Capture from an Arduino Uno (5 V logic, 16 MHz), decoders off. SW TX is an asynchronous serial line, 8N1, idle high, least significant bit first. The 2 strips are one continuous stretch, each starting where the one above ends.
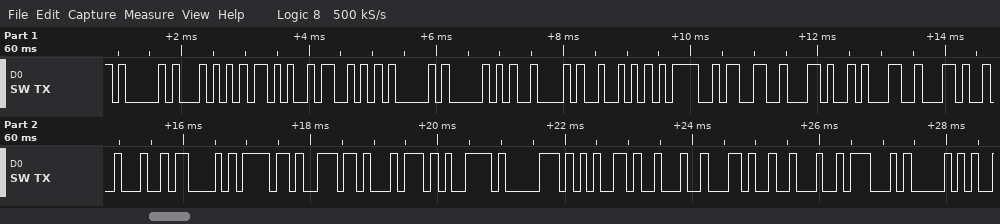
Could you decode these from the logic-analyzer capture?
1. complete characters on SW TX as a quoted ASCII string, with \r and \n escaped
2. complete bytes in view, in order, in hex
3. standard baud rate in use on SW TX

"AT+SAPBR=3,1,\"Contype\",\"GP"
0x41 0x54 0x2B 0x53 0x41 0x50 0x42 0x52 0x3D 0x33 0x2C 0x31 0x2C 0x22 0x43 0x6F 0x6E 0x74 0x79 0x70 0x65 0x22 0x2C 0x22 0x47 0x50
9600 baud
